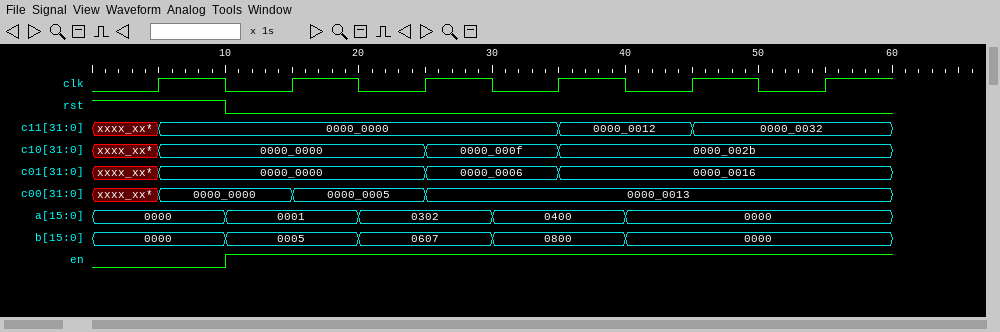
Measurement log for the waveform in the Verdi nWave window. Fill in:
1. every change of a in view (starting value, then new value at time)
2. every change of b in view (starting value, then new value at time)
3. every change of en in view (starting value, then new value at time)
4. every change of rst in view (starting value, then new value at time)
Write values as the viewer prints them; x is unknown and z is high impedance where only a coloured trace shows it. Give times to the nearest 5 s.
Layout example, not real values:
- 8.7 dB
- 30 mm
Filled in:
- 0000, 0001 at 10 s, 0302 at 20 s, 0400 at 30 s, 0000 at 40 s
- 0000, 0005 at 10 s, 0607 at 20 s, 0800 at 30 s, 0000 at 40 s
- 0, 1 at 10 s
- 1, 0 at 10 s
